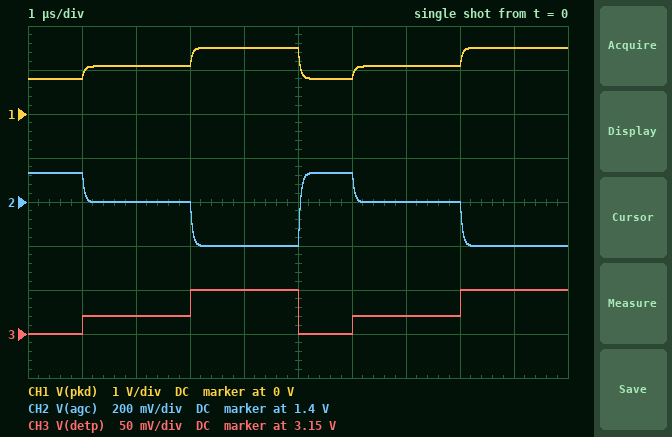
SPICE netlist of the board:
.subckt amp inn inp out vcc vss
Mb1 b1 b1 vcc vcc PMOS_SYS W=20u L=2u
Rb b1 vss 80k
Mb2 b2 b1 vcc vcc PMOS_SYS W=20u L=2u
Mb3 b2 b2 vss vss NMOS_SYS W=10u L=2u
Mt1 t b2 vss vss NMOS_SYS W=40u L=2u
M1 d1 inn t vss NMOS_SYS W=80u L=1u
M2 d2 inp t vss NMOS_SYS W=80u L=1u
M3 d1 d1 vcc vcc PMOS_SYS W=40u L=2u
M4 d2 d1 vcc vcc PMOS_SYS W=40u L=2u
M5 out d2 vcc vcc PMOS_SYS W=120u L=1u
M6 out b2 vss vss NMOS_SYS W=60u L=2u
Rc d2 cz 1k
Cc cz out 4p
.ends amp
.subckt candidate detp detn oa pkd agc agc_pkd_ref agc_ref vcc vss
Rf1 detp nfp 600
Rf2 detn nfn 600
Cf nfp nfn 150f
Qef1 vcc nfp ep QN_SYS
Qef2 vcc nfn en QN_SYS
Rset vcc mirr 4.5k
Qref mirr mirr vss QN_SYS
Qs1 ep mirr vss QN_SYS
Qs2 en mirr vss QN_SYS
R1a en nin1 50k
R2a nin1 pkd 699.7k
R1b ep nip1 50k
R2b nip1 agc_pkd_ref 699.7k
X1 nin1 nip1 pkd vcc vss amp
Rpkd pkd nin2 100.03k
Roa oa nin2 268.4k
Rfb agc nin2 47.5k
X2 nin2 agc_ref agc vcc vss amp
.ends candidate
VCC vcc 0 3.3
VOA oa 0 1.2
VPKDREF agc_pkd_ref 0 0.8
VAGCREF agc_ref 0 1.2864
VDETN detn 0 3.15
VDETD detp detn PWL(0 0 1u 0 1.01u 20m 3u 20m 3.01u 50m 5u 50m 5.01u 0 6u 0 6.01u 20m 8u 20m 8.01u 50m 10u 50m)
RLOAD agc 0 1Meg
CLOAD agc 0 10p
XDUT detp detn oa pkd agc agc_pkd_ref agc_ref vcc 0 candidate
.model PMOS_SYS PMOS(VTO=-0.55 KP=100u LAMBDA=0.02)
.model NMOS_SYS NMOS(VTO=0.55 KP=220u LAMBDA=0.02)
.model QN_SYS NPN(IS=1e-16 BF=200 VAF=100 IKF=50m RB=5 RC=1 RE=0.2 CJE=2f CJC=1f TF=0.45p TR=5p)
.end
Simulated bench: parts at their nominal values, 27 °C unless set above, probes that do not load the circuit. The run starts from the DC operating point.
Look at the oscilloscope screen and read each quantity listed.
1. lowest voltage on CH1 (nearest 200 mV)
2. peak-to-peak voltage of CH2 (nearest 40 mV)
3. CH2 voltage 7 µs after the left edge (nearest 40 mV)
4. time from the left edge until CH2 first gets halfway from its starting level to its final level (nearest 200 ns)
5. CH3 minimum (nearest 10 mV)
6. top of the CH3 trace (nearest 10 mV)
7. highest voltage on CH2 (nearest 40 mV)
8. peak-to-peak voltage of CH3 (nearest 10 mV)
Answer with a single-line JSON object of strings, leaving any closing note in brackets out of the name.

{"lowest voltage on CH1": "800 mV", "peak-to-peak voltage of CH2": "320 mV", "CH2 voltage 7 µs after the left edge": "1.40 V", "time from the left edge until CH2 first gets halfway from its starting level to its final level": "3.0 µs", "CH3 minimum": "3.15 V", "top of the CH3 trace": "3.20 V", "highest voltage on CH2": "1.52 V", "peak-to-peak voltage of CH3": "50 mV"}
